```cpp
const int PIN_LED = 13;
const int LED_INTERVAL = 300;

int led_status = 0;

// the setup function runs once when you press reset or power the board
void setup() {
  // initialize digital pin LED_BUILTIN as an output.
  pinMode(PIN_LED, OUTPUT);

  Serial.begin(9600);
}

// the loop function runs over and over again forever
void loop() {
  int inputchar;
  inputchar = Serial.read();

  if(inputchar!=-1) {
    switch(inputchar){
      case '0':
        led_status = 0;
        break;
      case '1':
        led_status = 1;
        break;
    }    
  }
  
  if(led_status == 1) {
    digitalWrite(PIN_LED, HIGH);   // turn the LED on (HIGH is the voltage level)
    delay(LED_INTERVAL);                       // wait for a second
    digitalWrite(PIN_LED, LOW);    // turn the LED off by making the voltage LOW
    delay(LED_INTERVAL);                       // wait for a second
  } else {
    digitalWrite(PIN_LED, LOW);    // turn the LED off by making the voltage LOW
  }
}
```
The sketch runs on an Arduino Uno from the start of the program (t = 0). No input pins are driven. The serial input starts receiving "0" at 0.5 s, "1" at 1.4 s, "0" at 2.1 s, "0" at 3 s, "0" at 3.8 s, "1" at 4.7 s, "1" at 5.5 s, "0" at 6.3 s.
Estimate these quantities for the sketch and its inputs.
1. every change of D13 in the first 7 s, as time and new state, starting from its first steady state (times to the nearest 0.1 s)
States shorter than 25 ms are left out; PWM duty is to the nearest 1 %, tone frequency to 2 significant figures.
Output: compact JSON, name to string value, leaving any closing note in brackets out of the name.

{"every change of D13 in the first 7 s, as time and new state, starting from its first steady state": "0 s low; 1.4 s high; 1.7 s low; 2 s high; 2.3 s low; 4.7 s high; 5 s low; 5.3 s high; 5.6 s low; 5.9 s high; 6.2 s low"}
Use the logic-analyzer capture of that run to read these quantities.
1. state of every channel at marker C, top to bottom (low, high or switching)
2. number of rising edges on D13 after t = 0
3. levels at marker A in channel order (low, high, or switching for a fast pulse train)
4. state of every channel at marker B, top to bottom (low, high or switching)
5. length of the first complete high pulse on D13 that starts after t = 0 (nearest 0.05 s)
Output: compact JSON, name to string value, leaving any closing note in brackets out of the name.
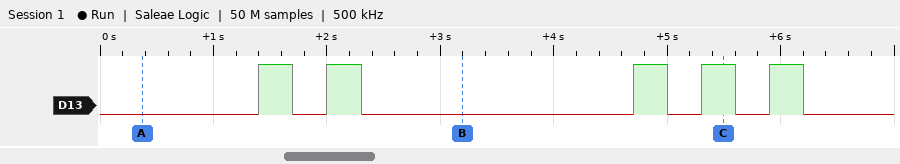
{"state of every channel at marker C, top to bottom": "D13 high", "number of rising edges on D13 after t = 0": "5", "levels at marker A in channel order": "D13 low", "state of every channel at marker B, top to bottom": "D13 low", "length of the first complete high pulse on D13 that starts after t = 0": "0.30 s"}
